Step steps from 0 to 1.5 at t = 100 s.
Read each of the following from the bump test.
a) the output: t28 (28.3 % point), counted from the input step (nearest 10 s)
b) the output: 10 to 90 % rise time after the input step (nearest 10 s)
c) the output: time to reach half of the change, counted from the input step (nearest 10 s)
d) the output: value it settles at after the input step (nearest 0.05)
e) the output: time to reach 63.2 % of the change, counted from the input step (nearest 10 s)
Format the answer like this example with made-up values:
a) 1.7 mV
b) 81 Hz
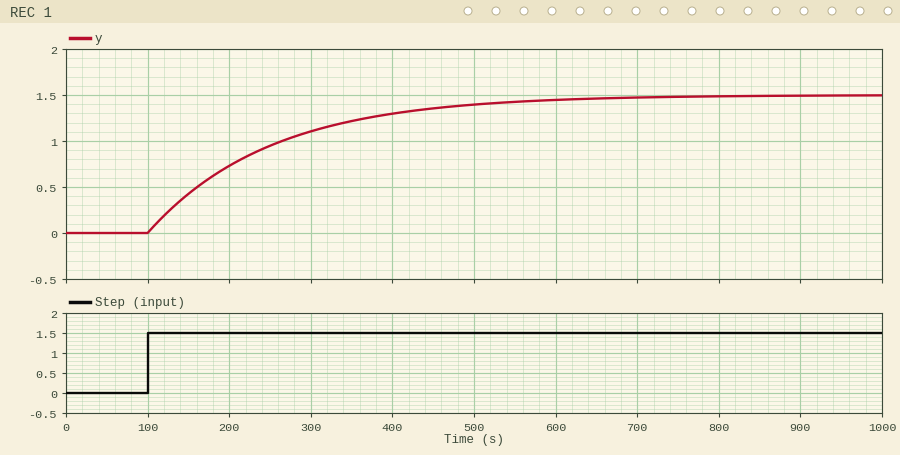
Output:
a) 50 s
b) 330 s
c) 100 s
d) 1.50
e) 150 s
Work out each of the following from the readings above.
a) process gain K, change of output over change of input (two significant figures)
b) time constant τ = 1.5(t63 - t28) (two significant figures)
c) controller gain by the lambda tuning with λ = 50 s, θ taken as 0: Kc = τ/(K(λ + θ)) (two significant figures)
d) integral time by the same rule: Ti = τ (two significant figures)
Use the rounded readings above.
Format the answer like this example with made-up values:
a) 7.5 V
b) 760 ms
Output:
a) 1.0
b) 150 s
c) 3.0
d) 150 s
